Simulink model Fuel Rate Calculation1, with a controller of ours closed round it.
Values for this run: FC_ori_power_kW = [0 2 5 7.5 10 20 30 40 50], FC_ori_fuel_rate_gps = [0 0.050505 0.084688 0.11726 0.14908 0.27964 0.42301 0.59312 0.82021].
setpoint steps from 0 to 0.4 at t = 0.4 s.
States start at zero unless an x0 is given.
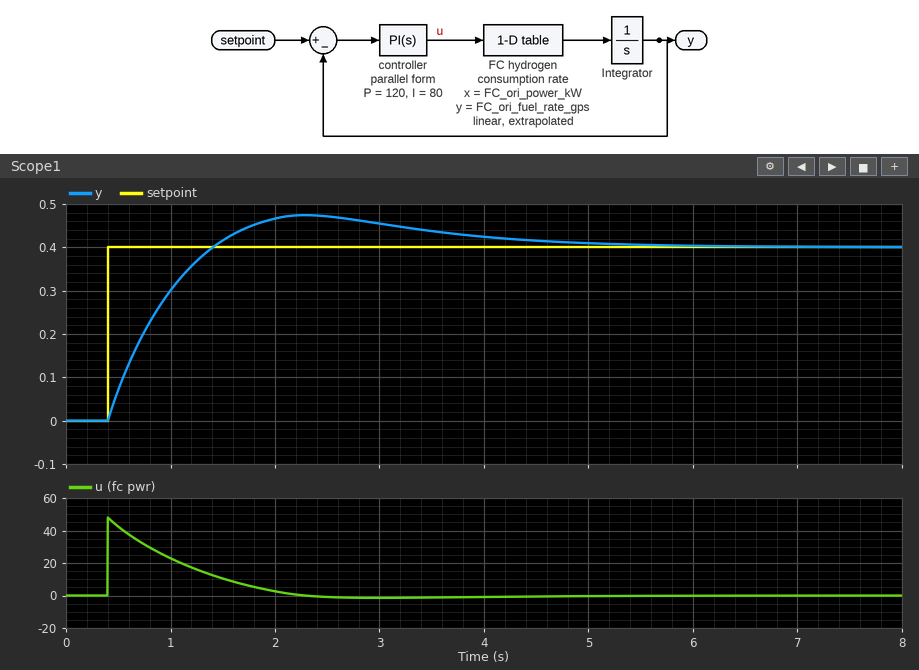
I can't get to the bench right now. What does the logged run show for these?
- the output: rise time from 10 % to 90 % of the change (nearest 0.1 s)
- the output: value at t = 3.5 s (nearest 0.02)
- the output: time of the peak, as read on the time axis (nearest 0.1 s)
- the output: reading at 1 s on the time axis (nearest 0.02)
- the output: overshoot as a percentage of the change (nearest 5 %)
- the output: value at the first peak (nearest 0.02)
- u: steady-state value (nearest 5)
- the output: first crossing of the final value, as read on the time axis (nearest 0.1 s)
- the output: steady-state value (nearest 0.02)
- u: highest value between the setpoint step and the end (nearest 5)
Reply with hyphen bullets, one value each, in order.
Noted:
- 0.8 s
- 0.44
- 2.3 s
- 0.30
- 20 %
- 0.48
- 0
- 1.4 s
- 0.40
- 50
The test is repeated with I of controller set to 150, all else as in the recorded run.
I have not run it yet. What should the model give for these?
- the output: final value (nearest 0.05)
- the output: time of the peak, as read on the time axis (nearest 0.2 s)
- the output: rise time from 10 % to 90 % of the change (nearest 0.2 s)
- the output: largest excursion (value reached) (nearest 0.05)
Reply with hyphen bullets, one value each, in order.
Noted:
- 0.40
- 2.0 s
- 0.6 s
- 0.50
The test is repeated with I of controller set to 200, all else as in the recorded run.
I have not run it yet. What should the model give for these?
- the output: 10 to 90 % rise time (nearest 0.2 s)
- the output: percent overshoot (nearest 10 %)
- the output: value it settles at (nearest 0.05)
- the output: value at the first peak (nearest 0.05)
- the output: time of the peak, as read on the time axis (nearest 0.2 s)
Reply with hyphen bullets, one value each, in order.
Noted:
- 0.6 s
- 30 %
- 0.40
- 0.50
- 1.8 s
